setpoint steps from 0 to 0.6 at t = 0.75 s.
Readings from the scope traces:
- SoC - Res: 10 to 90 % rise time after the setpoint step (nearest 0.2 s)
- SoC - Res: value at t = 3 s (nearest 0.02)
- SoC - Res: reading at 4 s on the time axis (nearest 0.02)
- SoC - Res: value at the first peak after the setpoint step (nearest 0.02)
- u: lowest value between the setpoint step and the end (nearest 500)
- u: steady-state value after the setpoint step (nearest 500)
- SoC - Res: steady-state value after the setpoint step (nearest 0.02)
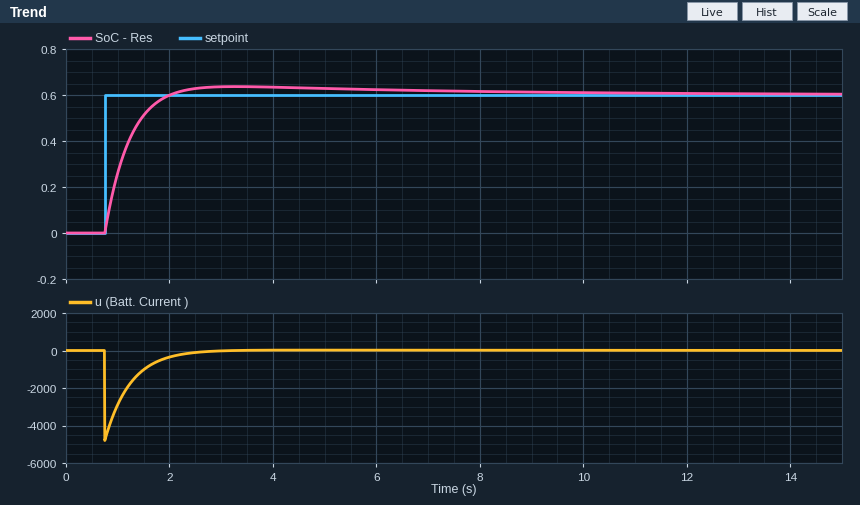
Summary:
0.8 s
0.64
0.64
0.64
-5000
0
0.60
